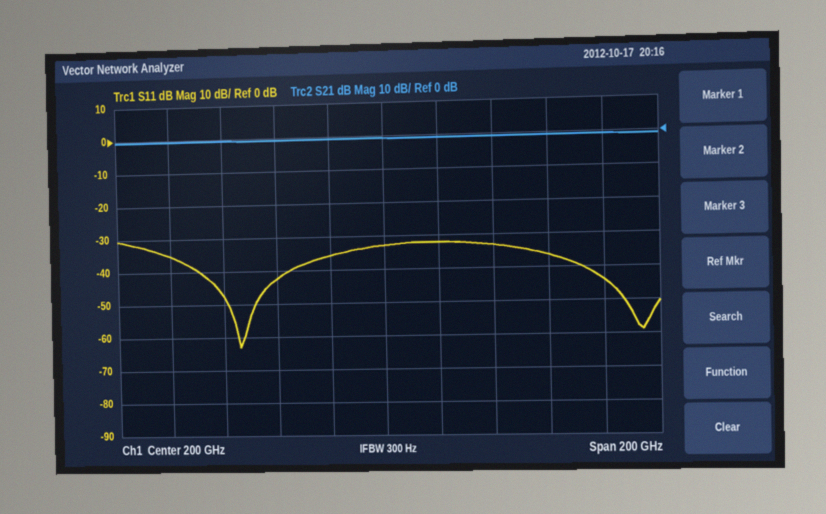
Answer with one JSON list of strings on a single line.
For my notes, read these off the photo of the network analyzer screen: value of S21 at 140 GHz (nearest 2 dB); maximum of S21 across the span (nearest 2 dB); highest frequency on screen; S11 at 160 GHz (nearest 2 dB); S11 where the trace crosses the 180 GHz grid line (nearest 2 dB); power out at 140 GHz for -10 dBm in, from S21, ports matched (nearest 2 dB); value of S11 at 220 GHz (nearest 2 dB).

["0 dB", "0 dB", "300 GHz", "-42 dB", "-36 dB", "-10 dBm", "-32 dB"]
